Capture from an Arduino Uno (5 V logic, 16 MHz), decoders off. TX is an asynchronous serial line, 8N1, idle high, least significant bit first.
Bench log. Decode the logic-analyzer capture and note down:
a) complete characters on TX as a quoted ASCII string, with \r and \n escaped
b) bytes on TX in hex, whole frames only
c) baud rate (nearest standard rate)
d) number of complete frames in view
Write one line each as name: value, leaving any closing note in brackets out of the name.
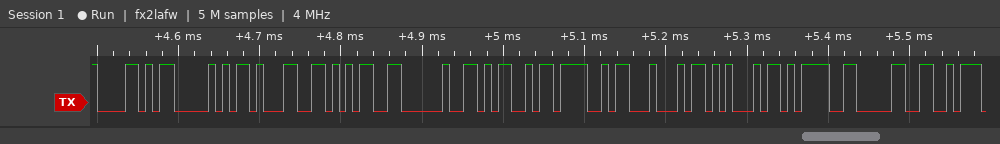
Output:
complete characters on TX as a quoted ASCII string, with \r and \n escaped: "XP15 MODE=0"
bytes on TX in hex, whole frames only: 0x58 0x50 0x31 0x35 0x20 0x4D 0x4F 0x44 0x45 0x3D 0x30
baud rate: 115200 baud
number of complete frames in view: 11
